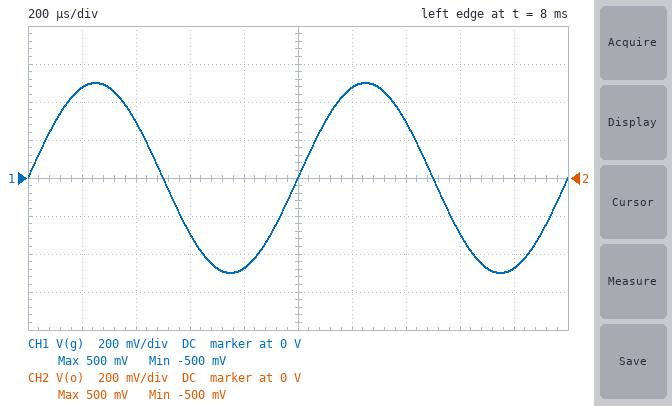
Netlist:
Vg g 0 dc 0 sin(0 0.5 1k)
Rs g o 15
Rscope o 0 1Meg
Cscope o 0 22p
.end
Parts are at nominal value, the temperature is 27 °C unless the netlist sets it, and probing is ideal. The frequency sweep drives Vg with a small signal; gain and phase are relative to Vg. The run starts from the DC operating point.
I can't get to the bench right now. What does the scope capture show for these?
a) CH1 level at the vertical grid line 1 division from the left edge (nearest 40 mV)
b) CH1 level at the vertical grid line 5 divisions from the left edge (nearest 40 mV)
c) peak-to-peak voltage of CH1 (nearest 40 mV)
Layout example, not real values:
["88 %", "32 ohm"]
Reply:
["480 mV", "0 V", "1.00 V"]
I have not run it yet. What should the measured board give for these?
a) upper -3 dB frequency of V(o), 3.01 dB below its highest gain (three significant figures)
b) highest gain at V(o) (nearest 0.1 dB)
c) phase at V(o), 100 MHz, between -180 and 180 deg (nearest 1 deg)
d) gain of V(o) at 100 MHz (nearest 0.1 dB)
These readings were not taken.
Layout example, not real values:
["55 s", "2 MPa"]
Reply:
["482 MHz", "0 dB", "-12 deg", "-0.2 dB"]
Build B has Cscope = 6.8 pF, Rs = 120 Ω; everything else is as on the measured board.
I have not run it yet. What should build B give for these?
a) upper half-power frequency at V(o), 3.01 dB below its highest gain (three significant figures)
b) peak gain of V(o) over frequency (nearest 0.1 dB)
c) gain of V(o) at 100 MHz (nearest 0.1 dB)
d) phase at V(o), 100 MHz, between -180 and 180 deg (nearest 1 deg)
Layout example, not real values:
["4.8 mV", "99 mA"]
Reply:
["195 MHz", "0 dB", "-1.0 dB", "-27 deg"]
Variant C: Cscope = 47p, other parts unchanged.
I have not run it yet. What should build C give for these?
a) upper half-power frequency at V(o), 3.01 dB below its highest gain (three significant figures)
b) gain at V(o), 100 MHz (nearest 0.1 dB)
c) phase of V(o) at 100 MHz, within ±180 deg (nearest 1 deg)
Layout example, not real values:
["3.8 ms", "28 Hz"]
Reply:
["226 MHz", "-0.8 dB", "-24 deg"]
